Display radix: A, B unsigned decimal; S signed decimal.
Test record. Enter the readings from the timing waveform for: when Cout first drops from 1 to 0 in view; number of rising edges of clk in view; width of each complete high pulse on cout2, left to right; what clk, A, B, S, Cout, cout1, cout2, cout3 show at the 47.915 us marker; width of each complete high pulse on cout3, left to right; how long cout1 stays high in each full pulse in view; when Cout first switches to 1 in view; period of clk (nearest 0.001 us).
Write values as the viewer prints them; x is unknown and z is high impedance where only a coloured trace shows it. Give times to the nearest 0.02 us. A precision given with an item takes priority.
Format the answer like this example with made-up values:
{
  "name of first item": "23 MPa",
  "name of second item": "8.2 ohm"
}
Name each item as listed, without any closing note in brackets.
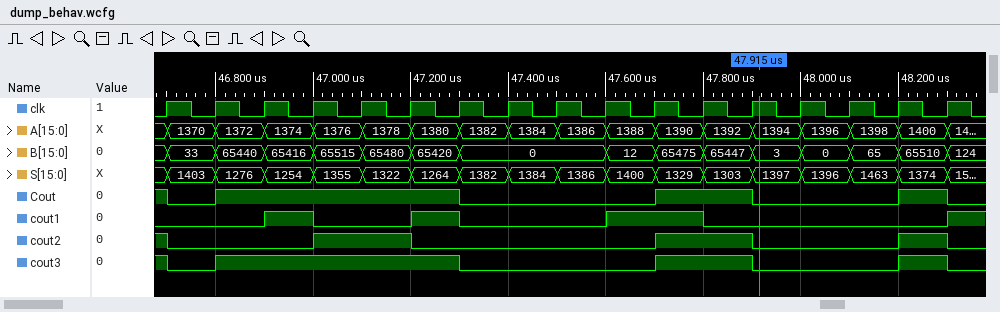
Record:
{
  "when Cout first drops from 1 to 0 in view": "46.7 us",
  "number of rising edges of clk in view": "17",
  "width of each complete high pulse on cout2, left to right": "0.2 us, 0.2 us, 0.1 us",
  "what clk, A, B, S, Cout, cout1, cout2, cout3 show at the 47.915 us marker": "clk=1, A=1394, B=3, S=1397, Cout=0, cout1=0, cout2=0, cout3=0",
  "width of each complete high pulse on cout3, left to right": "0.5 us, 0.2 us, 0.1 us",
  "how long cout1 stays high in each full pulse in view": "0.1 us, 0.1 us, 0.2 us",
  "when Cout first switches to 1 in view": "46.8 us",
  "period of clk": "0.1 us"
}
